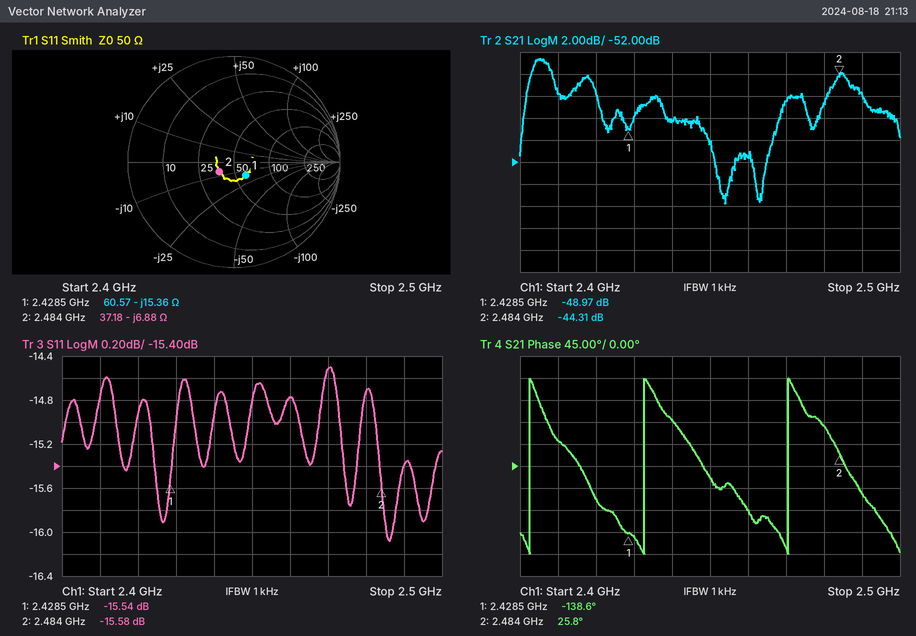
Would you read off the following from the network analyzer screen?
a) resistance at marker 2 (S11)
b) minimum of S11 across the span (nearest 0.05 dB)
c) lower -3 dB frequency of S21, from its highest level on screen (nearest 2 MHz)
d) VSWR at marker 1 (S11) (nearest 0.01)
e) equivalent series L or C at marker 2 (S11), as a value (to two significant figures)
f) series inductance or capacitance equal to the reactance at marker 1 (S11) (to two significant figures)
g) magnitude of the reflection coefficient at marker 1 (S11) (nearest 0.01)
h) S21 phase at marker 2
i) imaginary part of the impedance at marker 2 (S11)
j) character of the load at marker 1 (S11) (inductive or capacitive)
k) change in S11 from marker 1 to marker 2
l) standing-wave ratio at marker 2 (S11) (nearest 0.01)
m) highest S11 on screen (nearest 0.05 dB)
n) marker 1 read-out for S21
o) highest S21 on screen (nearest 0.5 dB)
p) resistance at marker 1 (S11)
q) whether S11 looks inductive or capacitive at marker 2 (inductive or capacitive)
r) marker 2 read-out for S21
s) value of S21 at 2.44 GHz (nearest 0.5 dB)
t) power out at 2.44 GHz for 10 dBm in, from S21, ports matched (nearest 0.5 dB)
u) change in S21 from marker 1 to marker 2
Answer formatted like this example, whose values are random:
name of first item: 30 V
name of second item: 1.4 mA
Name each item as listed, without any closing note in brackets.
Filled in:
resistance at marker 2: 37.18 Ω
minimum of S11 across the span: -16.10 dB
lower -3 dB frequency of S21, from its highest level on screen: 2.402 GHz
VSWR at marker 1 (S11): 1.40
equivalent series L or C at marker 2 (S11), as a value: 9.3 pF
series inductance or capacitance equal to the reactance at marker 1 (S11): 4.3 pF
magnitude of the reflection coefficient at marker 1 (S11): 0.17
S21 phase at marker 2: 25.8°
imaginary part of the impedance at marker 2: -6.88 Ω
character of the load at marker 1 (S11): capacitive
change in S11 from marker 1 to marker 2: -0.04 dB
standing-wave ratio at marker 2 (S11): 1.40
highest S11 on screen: -14.50 dB
marker 1 read-out for S21: -48.97 dB
highest S21 on screen: -42.5 dB
resistance at marker 1: 60.57 Ω
whether S11 looks inductive or capacitive at marker 2: capacitive
marker 2 read-out for S21: -44.31 dB
value of S21 at 2.44 GHz: -48.0 dB
power out at 2.44 GHz for 10 dBm in, from S21, ports matched: -38.0 dBm
change in S21 from marker 1 to marker 2: 4.66 dB
